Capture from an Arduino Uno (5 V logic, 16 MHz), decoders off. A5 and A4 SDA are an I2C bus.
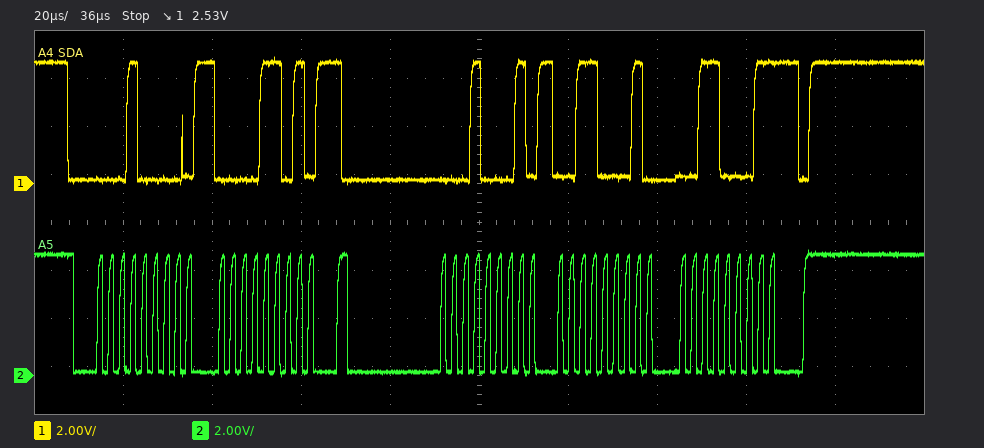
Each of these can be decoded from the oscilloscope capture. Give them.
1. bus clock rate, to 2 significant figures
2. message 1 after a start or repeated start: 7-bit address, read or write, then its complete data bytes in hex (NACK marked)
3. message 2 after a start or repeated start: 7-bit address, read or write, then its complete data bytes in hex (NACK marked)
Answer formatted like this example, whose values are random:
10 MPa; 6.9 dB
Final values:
400 kHz; 0x08 write: 0D; 0x08 read: 31 31 NACK
